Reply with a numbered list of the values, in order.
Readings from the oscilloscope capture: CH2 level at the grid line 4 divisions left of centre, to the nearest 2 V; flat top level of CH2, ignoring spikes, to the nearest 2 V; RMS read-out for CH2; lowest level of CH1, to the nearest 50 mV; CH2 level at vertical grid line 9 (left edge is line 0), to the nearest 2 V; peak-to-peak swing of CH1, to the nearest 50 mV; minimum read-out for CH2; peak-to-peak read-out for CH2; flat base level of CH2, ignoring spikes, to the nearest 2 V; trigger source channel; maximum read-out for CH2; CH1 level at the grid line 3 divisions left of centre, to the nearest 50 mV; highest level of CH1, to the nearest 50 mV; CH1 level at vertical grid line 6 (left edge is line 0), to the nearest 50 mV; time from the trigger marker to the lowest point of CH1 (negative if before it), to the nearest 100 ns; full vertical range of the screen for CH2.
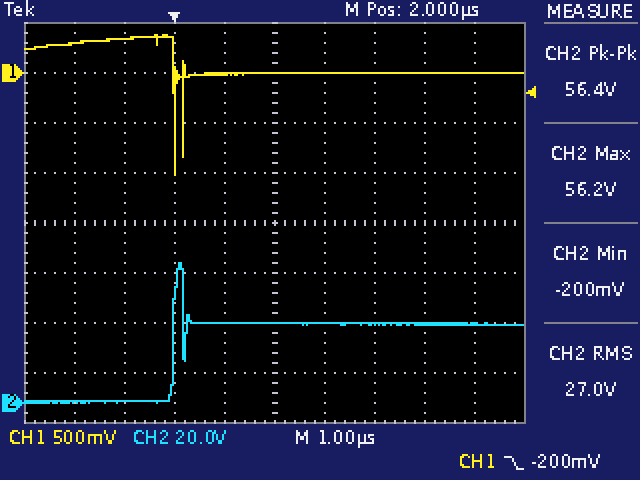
1. 0 V
2. 32 V
3. 27.0 V
4. -1.00 V
5. 32 V
6. 1.40 V
7. -200 mV
8. 56.4 V
9. 0 V
10. CH1
11. 56.2 V
12. 350 mV
13. 400 mV
14. 0 mV
15. 0.0 µs
16. 160 V
